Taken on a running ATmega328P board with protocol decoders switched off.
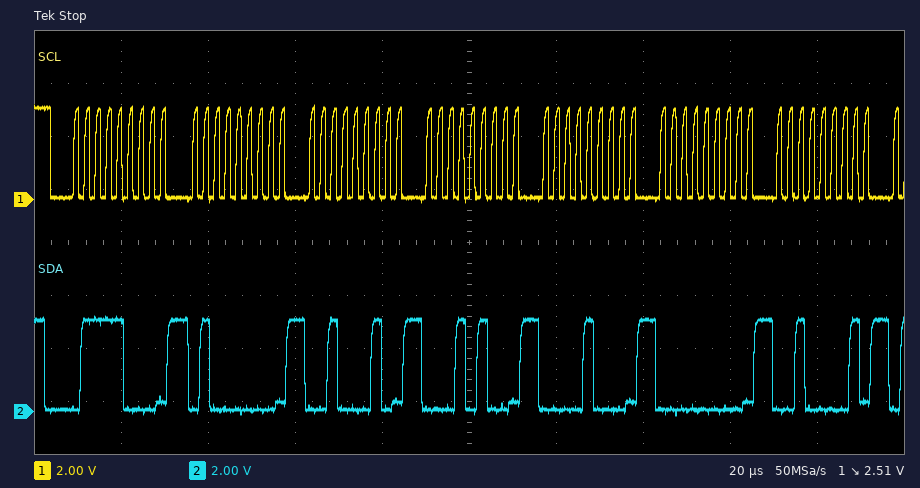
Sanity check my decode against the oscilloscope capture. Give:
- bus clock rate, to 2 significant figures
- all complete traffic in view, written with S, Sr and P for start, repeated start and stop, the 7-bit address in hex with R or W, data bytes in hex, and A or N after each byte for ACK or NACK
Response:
400 kHz
S 3CW A 40 A 22 A 14 A 08 A 00 A 21 A
